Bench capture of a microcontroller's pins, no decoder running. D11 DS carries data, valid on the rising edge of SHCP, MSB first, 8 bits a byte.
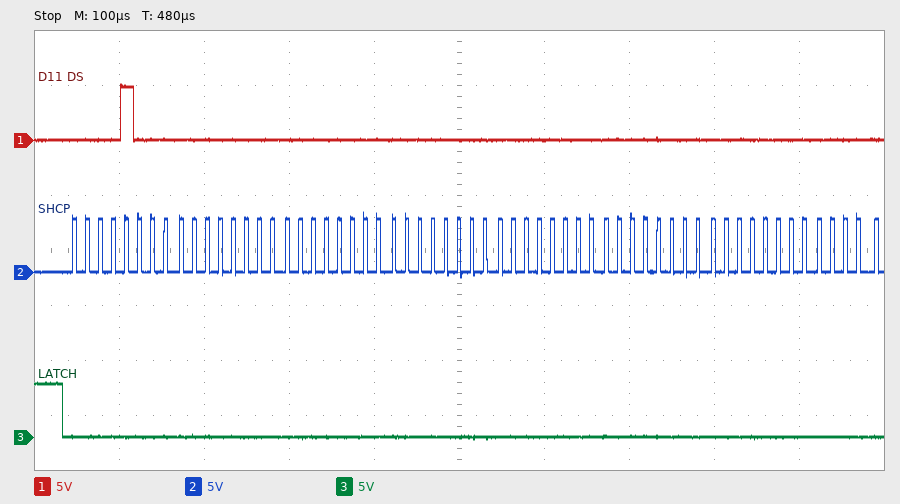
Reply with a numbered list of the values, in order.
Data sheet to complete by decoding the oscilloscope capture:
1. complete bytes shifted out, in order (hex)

1. 0x08 0x00 0x00 0x00 0x00 0x00 0x00
